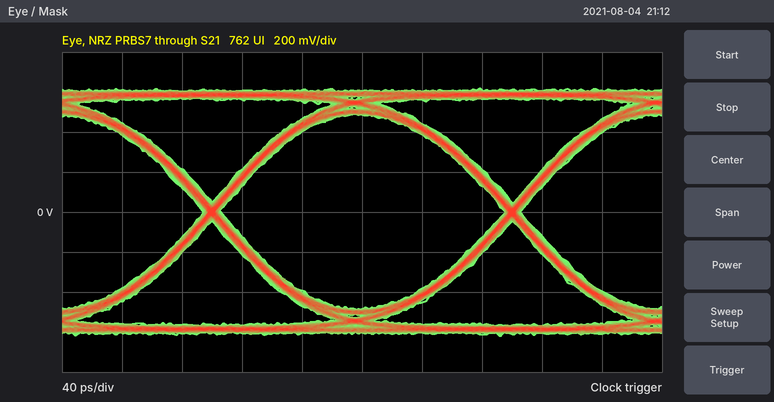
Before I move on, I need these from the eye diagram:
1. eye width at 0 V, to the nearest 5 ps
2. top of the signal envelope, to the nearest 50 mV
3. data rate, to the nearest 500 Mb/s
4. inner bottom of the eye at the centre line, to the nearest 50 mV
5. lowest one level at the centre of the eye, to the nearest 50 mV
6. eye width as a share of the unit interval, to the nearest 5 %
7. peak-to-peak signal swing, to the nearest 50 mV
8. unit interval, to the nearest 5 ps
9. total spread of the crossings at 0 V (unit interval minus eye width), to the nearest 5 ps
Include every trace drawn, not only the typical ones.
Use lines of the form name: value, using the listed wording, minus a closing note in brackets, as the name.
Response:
eye width at 0 V, to the nearest 5 ps: 190 ps
top of the signal envelope, to the nearest 50 mV: 600 mV
data rate, to the nearest 500 Mb/s: 5.0 Gb/s
inner bottom of the eye at the centre line, to the nearest 50 mV: -500 mV
lowest one level at the centre of the eye, to the nearest 50 mV: 500 mV
eye width as a share of the unit interval, to the nearest 5 %: 95 %
peak-to-peak signal swing, to the nearest 50 mV: 1.25 V
unit interval, to the nearest 5 ps: 200 ps
total spread of the crossings at 0 V (unit interval minus eye width), to the nearest 5 ps: 10 ps
